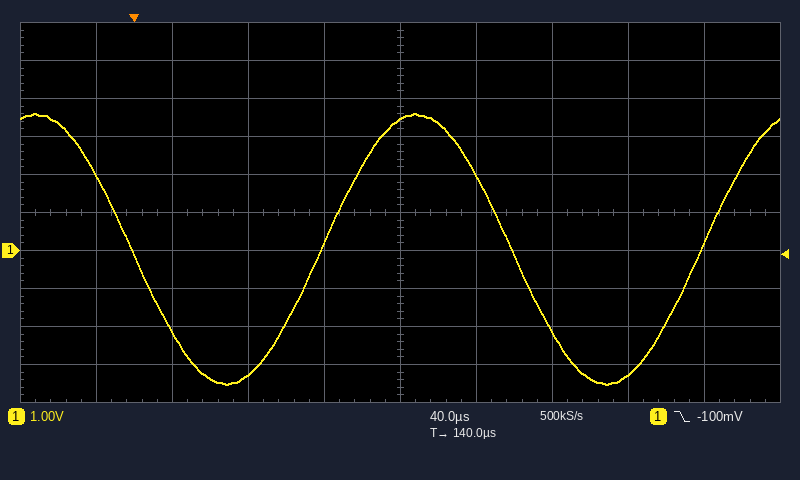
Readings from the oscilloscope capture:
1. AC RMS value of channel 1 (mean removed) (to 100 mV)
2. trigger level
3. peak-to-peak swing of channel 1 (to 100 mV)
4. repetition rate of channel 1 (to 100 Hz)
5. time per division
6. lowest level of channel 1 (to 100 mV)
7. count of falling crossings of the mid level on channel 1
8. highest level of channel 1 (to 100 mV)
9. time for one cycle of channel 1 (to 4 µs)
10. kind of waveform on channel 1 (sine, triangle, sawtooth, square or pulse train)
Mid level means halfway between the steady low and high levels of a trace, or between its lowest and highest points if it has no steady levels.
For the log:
2.5 V
-100 mV
7.1 V
5.0 kHz
40 µs
-3.5 V
2
3.6 V
200 µs
sine
